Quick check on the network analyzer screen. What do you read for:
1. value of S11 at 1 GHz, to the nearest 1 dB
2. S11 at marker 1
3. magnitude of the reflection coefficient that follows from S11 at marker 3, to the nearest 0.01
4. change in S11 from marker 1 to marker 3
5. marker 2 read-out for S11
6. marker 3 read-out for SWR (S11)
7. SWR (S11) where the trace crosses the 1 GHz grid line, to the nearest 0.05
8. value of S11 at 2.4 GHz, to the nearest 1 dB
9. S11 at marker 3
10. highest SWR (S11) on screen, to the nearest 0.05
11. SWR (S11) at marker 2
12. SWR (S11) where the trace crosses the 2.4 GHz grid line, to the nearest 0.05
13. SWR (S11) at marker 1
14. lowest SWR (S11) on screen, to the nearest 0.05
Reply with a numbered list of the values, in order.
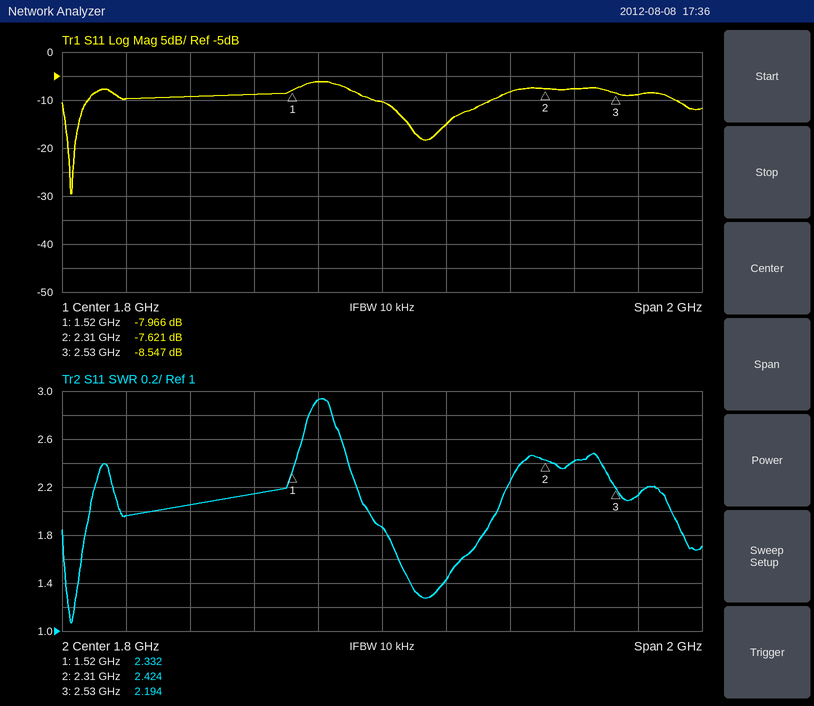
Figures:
1. -10 dB
2. -7.966 dB
3. 0.37
4. -0.581 dB
5. -7.621 dB
6. 2.194
7. 1.95
8. -8 dB
9. -8.547 dB
10. 2.95
11. 2.424
12. 2.40
13. 2.332
14. 1.05
